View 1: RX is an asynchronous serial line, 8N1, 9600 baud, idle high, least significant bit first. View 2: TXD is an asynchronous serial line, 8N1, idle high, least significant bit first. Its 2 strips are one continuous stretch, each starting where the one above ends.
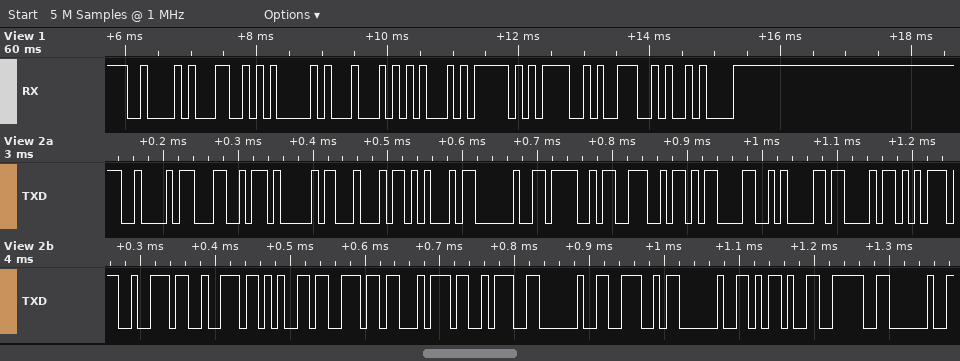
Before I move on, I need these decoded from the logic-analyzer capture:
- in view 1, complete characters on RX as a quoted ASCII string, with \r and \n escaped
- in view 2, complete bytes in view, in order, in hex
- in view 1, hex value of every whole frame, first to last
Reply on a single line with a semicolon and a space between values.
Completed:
"BLADE_ON\n"; 0x42 0x4C 0x41 0x44 0x45 0x20 0x4F 0x4E 0x0D 0x0A 0x43 0x75 0x72 0x72 0x65 0x6E 0x74 0x3A 0x20 0x4E 0x20 0x2D 0x3E 0x20; 42 4C 41 44 45 5F 4F 4E 0A
